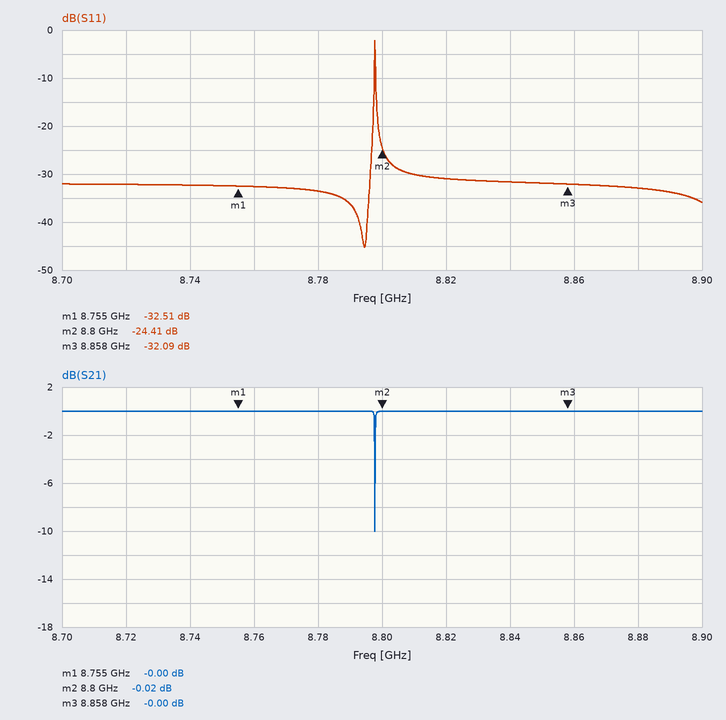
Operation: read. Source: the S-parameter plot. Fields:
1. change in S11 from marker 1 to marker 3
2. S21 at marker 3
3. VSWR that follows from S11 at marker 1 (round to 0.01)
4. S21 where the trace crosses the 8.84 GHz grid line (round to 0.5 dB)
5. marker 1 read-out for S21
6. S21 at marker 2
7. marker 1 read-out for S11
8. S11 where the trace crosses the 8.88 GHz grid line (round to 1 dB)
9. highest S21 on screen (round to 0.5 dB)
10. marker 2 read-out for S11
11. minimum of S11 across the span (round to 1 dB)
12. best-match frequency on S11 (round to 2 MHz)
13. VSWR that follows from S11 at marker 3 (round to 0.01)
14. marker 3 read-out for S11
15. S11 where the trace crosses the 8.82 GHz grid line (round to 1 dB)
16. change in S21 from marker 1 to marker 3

0.42 dB
-0.00 dB
1.05
0.0 dB
-0.00 dB
-0.02 dB
-32.51 dB
-33 dB
0.0 dB
-24.41 dB
-45 dB
8.794 GHz
1.05
-32.09 dB
-31 dB
0.00 dB
